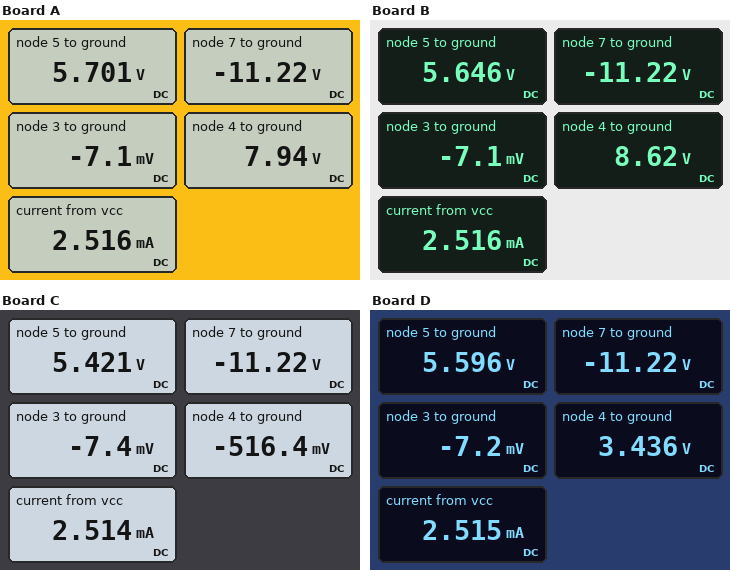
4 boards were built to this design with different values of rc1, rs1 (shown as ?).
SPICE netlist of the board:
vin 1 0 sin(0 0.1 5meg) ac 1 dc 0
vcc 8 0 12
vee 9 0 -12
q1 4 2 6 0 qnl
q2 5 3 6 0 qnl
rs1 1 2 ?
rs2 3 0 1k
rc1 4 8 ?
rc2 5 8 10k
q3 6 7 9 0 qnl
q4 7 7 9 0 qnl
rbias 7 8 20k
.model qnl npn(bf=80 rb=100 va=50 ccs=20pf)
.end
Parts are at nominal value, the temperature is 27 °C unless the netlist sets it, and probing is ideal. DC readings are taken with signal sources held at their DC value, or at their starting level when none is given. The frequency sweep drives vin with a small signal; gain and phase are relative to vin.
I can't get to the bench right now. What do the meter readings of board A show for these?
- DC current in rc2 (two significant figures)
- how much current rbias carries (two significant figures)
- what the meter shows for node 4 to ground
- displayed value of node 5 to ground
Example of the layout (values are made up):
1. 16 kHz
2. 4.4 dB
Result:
1. 630 µA
2. 1.2 mA
3. 7.94 V
4. 5.701 V
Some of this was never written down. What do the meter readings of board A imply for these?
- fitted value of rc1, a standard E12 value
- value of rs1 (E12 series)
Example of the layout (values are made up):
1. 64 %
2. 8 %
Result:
1. 5.6 kΩ
2. 560 Ω
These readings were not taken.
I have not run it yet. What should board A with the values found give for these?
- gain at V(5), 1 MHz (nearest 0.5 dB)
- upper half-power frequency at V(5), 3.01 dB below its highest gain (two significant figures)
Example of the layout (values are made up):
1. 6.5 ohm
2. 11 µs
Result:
1. 36.0 dB
2. 860 kHz
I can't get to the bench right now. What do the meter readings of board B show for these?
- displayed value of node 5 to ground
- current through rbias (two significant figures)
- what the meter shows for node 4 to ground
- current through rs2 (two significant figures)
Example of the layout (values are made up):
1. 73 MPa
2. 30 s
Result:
1. 5.646 V
2. 1.2 mA
3. 8.62 V
4. 7.1 µA
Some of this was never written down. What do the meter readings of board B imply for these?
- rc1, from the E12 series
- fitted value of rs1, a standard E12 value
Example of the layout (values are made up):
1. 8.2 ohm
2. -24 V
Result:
1. 4.7 kΩ
2. 680 Ω
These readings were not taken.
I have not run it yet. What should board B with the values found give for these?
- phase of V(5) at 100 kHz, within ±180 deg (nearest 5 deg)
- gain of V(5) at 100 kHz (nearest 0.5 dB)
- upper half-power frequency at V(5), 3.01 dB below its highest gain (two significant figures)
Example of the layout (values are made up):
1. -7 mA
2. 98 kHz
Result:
1. -5 deg
2. 39.5 dB
3. 850 kHz
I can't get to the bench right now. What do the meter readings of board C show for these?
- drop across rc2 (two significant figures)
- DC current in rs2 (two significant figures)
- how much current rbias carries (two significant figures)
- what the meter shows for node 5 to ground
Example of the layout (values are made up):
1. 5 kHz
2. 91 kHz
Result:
1. 6.6 V
2. 7.4 µA
3. 1.2 mA
4. 5.421 V
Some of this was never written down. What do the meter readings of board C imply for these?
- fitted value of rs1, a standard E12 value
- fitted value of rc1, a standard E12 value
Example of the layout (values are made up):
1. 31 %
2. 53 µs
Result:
1. 330 Ω
2. 18 kΩ
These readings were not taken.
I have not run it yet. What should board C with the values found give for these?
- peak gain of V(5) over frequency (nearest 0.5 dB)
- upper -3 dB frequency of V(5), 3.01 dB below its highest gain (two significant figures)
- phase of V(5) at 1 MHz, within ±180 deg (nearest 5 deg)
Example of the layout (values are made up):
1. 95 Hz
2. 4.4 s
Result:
1. 38.0 dB
2. 1.1 MHz
3. -45 deg
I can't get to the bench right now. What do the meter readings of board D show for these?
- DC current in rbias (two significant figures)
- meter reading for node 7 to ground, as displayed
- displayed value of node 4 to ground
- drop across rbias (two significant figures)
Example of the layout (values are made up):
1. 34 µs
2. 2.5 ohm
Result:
1. 1.2 mA
2. -11.22 V
3. 3.436 V
4. 23 V
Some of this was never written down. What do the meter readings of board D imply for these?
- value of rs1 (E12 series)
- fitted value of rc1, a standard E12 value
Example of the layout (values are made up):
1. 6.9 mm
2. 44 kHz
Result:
1. 390 Ω
2. 12 kΩ
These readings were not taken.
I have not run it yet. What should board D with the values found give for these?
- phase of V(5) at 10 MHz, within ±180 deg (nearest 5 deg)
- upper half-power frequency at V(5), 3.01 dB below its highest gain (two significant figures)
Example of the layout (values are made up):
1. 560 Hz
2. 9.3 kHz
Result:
1. -85 deg
2. 910 kHz
